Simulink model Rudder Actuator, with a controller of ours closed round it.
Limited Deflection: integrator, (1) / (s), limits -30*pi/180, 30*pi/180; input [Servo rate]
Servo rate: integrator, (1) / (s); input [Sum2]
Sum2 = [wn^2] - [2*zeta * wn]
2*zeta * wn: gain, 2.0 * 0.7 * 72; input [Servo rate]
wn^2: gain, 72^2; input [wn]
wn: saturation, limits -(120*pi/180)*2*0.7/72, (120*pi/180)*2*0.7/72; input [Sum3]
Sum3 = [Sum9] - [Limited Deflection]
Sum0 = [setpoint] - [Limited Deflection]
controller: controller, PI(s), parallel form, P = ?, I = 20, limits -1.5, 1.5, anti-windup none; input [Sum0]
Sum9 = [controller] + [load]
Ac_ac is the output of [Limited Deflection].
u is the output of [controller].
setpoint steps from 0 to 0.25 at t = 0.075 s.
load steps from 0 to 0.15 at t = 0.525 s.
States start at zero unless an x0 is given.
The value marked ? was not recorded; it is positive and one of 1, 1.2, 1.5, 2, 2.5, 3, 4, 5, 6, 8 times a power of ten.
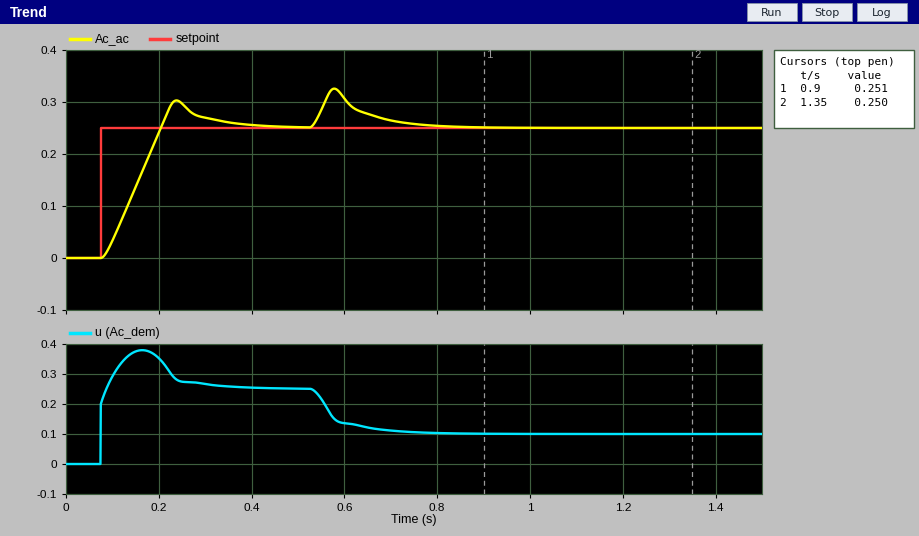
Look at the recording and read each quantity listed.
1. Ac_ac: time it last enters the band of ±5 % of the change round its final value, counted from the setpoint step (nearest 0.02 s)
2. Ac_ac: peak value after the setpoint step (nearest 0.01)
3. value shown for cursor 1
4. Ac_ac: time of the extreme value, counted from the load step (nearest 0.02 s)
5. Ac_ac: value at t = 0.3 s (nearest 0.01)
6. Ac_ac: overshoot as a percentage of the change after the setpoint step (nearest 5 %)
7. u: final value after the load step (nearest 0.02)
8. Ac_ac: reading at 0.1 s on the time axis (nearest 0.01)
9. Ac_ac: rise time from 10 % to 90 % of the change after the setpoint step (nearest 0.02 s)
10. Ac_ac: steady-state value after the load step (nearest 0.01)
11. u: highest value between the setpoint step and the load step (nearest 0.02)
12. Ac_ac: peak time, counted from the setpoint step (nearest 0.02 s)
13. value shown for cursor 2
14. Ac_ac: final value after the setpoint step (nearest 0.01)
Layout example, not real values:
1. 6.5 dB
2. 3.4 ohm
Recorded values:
1. 0.26 s
2. 0.30
3. 0.251
4. 0.06 s
5. 0.27
6. 20 %
7. 0.10
8. 0.03
9. 0.10 s
10. 0.25
11. 0.38
12. 0.16 s
13. 0.250
14. 0.25
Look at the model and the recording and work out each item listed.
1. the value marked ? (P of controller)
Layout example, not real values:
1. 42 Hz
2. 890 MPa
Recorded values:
1. 0.8
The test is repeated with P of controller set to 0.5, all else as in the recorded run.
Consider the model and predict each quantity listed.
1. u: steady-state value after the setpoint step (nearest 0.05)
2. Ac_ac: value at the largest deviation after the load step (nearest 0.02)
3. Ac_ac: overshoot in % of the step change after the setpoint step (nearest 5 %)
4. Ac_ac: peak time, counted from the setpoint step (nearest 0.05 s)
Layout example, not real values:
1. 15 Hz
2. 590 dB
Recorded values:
1. 0.25
2. 0.34
3. 25 %
4. 0.15 s
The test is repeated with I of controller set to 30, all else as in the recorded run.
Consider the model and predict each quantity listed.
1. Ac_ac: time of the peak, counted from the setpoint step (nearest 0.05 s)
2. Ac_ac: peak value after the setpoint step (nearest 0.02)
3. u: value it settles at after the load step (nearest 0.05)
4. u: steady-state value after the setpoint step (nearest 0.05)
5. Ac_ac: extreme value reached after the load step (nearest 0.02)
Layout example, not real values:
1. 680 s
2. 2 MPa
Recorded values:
1. 0.20 s
2. 0.36
3. 0.10
4. 0.25
5. 0.32
